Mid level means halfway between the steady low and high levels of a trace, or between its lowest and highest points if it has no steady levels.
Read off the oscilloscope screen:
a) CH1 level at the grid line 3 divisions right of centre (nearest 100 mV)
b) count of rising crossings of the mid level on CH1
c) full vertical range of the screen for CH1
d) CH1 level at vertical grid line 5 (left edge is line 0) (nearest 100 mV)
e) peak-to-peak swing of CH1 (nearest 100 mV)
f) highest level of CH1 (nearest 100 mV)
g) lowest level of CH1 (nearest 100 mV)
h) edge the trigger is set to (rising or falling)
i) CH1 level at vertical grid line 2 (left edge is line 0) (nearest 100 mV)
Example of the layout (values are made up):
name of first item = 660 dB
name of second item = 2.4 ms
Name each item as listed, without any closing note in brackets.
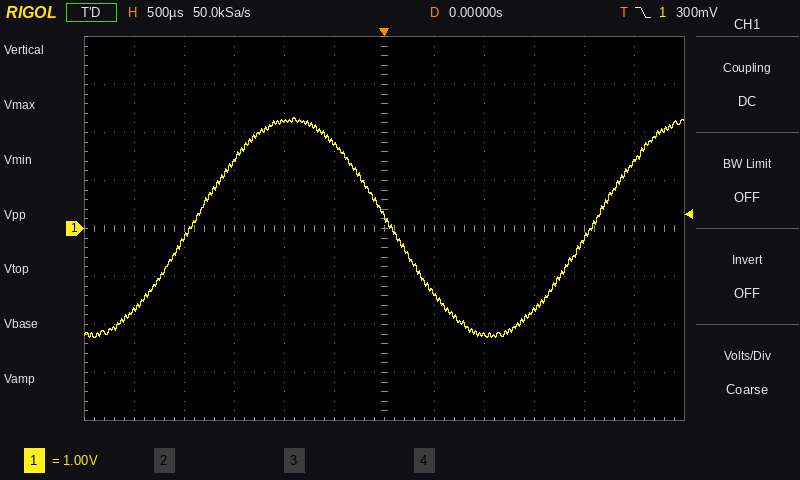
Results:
CH1 level at the grid line 3 divisions right of centre = -1.7 V
count of rising crossings of the mid level on CH1 = 2
full vertical range of the screen for CH1 = 8 V
CH1 level at vertical grid line 5 (left edge is line 0) = 1.8 V
peak-to-peak swing of CH1 = 4.6 V
highest level of CH1 = 2.3 V
lowest level of CH1 = -2.3 V
edge the trigger is set to = falling
CH1 level at vertical grid line 2 (left edge is line 0) = -200 mV
